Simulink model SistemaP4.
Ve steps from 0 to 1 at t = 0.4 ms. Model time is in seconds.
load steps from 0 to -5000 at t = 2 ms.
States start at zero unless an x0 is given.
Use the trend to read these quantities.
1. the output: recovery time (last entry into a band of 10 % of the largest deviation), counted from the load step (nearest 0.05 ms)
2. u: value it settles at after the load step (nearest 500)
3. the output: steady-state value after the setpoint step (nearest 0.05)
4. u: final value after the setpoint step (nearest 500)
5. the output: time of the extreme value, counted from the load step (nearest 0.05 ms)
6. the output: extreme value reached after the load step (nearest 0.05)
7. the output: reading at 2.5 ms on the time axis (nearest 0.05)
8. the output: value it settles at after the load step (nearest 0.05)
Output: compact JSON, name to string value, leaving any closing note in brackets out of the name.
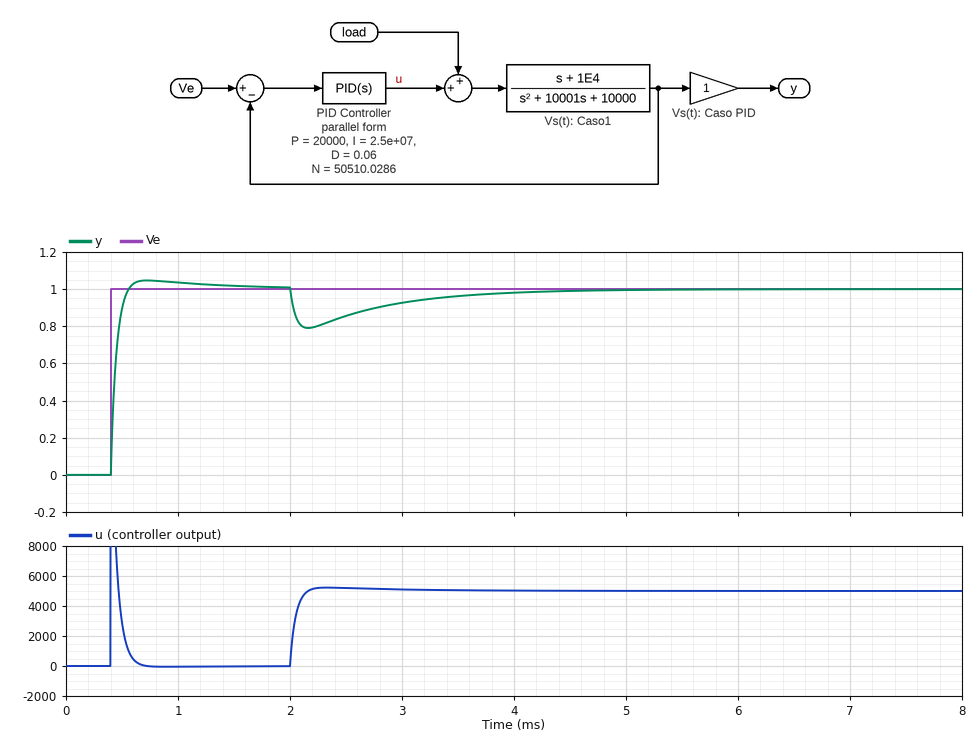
{"the output: recovery time (last entry into a band of 10 % of the largest deviation), counted from the load step": "1.90 ms", "u: value it settles at after the load step": "5000", "the output: steady-state value after the setpoint step": "1.00", "u: final value after the setpoint step": "0", "the output: time of the extreme value, counted from the load step": "0.15 ms", "the output: extreme value reached after the load step": "0.80", "the output: reading at 2.5 ms on the time axis": "0.85", "the output: value it settles at after the load step": "1.00"}
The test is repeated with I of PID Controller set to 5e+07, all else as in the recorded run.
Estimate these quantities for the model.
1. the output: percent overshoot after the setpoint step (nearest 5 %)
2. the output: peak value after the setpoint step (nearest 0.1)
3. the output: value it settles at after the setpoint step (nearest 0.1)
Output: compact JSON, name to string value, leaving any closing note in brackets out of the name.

{"the output: percent overshoot after the setpoint step": "10 %", "the output: peak value after the setpoint step": "1.1", "the output: value it settles at after the setpoint step": "1.0"}
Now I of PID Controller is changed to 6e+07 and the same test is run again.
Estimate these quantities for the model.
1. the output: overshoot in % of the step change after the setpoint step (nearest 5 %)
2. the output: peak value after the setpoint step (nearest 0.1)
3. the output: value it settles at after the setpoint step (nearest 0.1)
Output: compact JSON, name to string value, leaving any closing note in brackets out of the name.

{"the output: overshoot in % of the step change after the setpoint step": "10 %", "the output: peak value after the setpoint step": "1.1", "the output: value it settles at after the setpoint step": "1.0"}
